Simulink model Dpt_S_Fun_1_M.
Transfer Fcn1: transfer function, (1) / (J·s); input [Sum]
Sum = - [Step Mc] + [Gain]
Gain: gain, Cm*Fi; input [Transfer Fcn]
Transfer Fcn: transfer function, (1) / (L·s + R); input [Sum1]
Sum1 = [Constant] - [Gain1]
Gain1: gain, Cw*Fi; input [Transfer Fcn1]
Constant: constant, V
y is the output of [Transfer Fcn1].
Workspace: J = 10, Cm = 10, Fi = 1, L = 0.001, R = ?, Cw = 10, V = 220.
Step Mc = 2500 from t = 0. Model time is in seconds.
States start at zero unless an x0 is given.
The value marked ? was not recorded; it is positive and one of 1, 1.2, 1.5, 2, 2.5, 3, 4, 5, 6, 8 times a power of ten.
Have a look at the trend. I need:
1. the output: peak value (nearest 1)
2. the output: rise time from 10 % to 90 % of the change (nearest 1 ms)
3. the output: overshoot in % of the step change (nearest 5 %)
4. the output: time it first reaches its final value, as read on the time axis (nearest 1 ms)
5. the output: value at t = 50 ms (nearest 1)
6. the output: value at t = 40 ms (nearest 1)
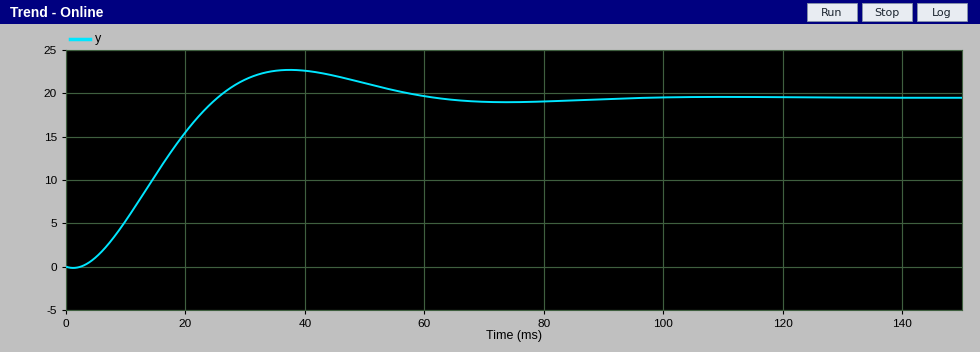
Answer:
23
16 ms
15 %
25 ms
21
23
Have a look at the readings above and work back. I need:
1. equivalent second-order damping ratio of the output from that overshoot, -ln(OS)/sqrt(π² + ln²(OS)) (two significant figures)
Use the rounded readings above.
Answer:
0.52
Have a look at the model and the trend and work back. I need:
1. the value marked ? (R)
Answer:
0.1
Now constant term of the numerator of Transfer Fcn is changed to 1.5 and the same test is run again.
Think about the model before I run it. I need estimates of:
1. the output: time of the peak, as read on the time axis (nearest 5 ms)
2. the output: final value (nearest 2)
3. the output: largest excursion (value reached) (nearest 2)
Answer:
30 ms
20
26
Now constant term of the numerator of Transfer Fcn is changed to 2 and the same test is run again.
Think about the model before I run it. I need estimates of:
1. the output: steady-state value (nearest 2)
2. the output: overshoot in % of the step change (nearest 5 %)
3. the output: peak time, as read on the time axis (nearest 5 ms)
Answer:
20
30 %
25 ms
